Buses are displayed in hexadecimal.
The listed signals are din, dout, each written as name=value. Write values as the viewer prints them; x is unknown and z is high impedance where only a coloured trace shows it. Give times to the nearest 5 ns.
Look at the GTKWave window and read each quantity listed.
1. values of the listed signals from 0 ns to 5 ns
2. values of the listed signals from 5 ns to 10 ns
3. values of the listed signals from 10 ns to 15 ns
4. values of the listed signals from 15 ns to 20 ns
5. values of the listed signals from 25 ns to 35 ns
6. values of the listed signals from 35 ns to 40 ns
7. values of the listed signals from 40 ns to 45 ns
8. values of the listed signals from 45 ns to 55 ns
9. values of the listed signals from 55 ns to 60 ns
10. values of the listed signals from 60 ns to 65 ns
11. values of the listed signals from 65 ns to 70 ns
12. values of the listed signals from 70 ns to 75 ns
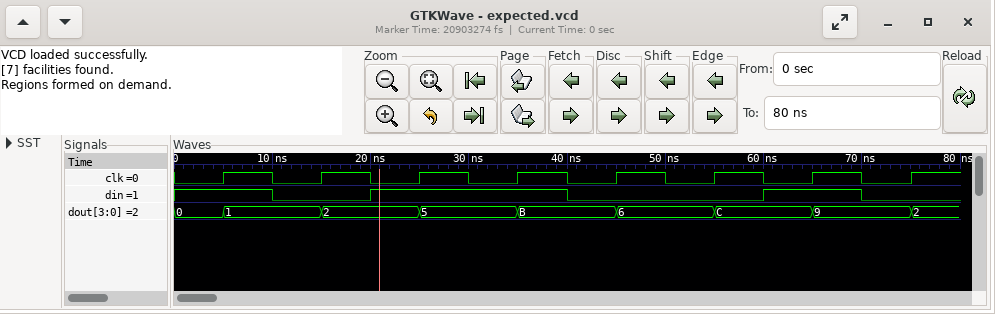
din=1, dout=0
din=1, dout=1
din=0, dout=1
din=0, dout=2
din=1, dout=5
din=1, dout=B
din=0, dout=B
din=0, dout=6
din=0, dout=C
din=1, dout=C
din=1, dout=9
din=0, dout=9
